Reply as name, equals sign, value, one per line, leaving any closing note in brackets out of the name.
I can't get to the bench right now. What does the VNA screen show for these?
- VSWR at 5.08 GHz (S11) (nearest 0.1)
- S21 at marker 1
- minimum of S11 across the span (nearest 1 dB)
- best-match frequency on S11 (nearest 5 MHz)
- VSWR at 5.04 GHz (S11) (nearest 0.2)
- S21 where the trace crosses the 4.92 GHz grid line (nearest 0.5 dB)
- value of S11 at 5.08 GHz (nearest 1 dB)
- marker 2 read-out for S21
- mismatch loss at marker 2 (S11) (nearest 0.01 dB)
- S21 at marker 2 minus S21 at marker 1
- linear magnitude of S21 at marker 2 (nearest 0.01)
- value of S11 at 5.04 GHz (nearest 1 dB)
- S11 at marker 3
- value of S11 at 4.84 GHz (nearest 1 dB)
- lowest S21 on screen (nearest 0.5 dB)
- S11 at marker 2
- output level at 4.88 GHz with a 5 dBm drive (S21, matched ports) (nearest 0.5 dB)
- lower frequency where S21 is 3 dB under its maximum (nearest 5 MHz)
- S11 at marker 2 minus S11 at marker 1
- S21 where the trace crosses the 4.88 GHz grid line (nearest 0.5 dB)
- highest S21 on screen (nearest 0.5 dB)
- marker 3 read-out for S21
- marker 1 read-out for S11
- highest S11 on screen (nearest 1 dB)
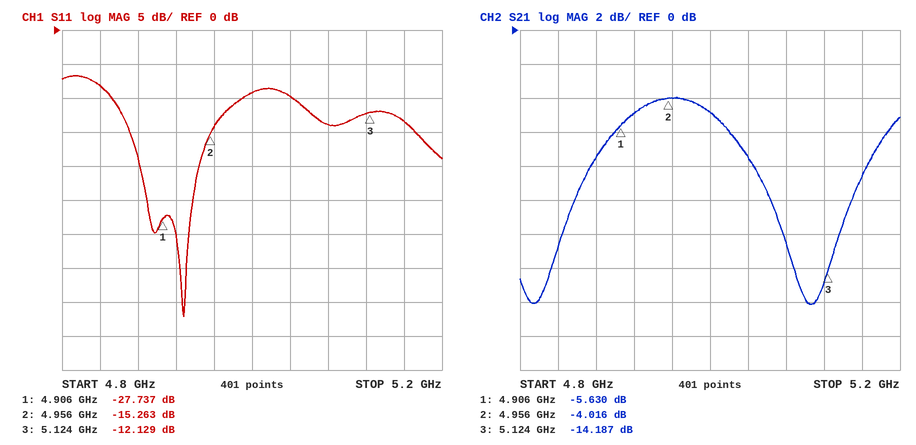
VSWR at 5.08 GHz (S11) = 1.5
S21 at marker 1 = -5.630 dB
minimum of S11 across the span = -42 dB
best-match frequency on S11 = 4.930 GHz
VSWR at 5.04 GHz (S11) = 2.0
S21 where the trace crosses the 4.92 GHz grid line = -5.0 dB
value of S11 at 5.08 GHz = -14 dB
marker 2 read-out for S21 = -4.016 dB
mismatch loss at marker 2 (S11) = 0.13 dB
S21 at marker 2 minus S21 at marker 1 = 1.614 dB
linear magnitude of S21 at marker 2 = 0.63
value of S11 at 5.04 GHz = -10 dB
S11 at marker 3 = -12.129 dB
value of S11 at 4.84 GHz = -8 dB
lowest S21 on screen = -16.0 dB
S11 at marker 2 = -15.263 dB
output level at 4.88 GHz with a 5 dBm drive (S21, matched ports) = -2.5 dBm
lower frequency where S21 is 3 dB under its maximum = 4.885 GHz
S11 at marker 2 minus S11 at marker 1 = 12.474 dB
S21 where the trace crosses the 4.88 GHz grid line = -7.5 dB
highest S21 on screen = -4.0 dB
marker 3 read-out for S21 = -14.187 dB
marker 1 read-out for S11 = -27.737 dB
highest S11 on screen = -7 dB
